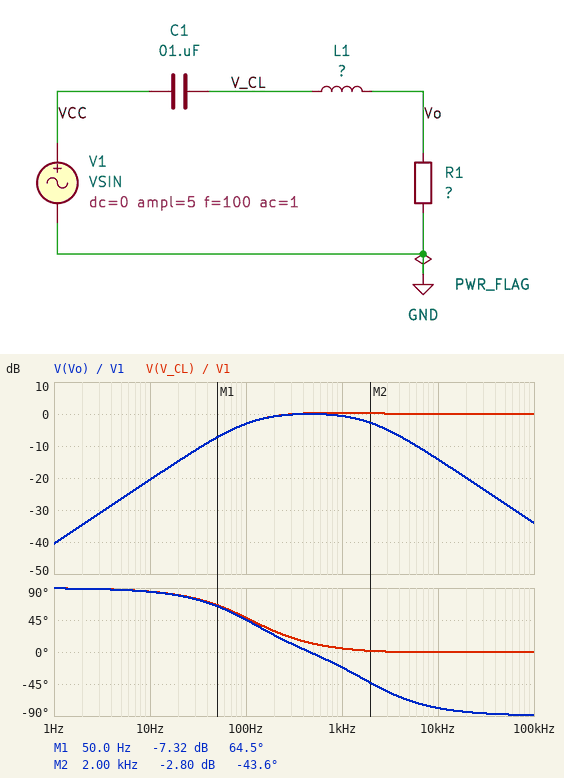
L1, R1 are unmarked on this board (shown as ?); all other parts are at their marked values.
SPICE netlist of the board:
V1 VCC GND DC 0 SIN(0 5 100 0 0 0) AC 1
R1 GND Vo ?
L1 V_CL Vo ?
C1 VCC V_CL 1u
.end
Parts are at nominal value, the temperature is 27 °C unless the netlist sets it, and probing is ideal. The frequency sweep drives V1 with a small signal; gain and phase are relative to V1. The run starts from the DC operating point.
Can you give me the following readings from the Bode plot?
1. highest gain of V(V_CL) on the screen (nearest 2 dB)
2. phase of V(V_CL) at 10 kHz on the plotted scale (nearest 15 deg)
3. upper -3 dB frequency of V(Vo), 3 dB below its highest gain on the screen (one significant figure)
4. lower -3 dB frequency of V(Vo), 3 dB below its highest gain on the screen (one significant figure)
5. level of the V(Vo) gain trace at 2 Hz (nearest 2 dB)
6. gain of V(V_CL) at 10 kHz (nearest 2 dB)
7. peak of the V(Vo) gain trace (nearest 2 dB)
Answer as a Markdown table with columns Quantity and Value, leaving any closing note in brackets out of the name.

| Quantity | Value |
|---|---|
| highest gain of V(V_CL) on the screen | 0 dB |
| phase of V(V_CL) at 10 kHz on the plotted scale | 0 deg |
| upper -3 dB frequency of V(Vo), 3 dB below its highest gain on the screen | 2 kHz |
| lower -3 dB frequency of V(Vo), 3 dB below its highest gain on the screen | 100 Hz |
| level of the V(Vo) gain trace at 2 Hz | -34 dB |
| gain of V(V_CL) at 10 kHz | 0 dB |
| peak of the V(Vo) gain trace | 0 dB |
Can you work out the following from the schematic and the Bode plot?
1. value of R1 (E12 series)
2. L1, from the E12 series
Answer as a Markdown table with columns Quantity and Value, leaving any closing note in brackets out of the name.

| Quantity | Value |
|---|---|
| value of R1 | 1.5 kΩ |
| L1, from the E12 series | 120 mH |
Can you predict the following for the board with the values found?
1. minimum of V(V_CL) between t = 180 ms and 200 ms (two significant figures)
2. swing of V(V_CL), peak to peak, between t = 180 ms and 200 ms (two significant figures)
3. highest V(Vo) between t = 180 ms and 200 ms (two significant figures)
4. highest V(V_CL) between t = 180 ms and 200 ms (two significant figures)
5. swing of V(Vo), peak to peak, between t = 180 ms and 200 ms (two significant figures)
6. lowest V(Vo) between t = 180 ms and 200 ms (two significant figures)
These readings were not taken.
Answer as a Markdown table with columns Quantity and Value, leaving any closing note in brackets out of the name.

| Quantity | Value |
|---|---|
| minimum of V(V_CL) between t = 180 ms and 200 ms | -3.5 V |
| swing of V(V_CL), peak to peak, between t = 180 ms and 200 ms | 7.0 V |
| highest V(Vo) between t = 180 ms and 200 ms | 3.5 V |
| highest V(V_CL) between t = 180 ms and 200 ms | 3.5 V |
| swing of V(Vo), peak to peak, between t = 180 ms and 200 ms | 7.0 V |
| lowest V(Vo) between t = 180 ms and 200 ms | -3.5 V |
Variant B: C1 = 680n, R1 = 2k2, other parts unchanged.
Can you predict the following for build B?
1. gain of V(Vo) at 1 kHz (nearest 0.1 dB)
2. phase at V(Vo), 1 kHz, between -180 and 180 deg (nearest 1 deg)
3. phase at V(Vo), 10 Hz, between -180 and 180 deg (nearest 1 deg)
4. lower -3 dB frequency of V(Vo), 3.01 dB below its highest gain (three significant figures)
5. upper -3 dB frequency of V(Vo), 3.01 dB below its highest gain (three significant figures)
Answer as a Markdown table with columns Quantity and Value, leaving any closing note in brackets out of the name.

| Quantity | Value |
|---|---|
| gain of V(Vo) at 1 kHz | -0.2 dB |
| phase at V(Vo), 1 kHz, between -180 and 180 deg | -13 deg |
| phase at V(Vo), 10 Hz, between -180 and 180 deg | 85 deg |
| lower -3 dB frequency of V(Vo), 3.01 dB below its highest gain | 103 Hz |
| upper -3 dB frequency of V(Vo), 3.01 dB below its highest gain | 3.02 kHz |
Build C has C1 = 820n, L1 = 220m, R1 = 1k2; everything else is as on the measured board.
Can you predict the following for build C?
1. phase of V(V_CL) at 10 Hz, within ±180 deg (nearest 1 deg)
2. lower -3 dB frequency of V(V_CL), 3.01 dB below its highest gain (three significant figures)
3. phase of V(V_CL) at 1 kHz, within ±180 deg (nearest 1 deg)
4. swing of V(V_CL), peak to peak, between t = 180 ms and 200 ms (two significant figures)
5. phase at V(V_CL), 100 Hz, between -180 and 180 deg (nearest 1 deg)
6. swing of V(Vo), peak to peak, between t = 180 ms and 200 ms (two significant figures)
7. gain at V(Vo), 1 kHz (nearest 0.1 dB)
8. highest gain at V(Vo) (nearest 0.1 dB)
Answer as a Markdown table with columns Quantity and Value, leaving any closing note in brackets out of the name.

| Quantity | Value |
|---|---|
| phase of V(V_CL) at 10 Hz, within ±180 deg | 87 deg |
| lower -3 dB frequency of V(V_CL), 3.01 dB below its highest gain | 163 Hz |
| phase of V(V_CL) at 1 kHz, within ±180 deg | 4 deg |
| swing of V(V_CL), peak to peak, between t = 180 ms and 200 ms | 5.6 V |
| phase at V(V_CL), 100 Hz, between -180 and 180 deg | 63 deg |
| swing of V(Vo), peak to peak, between t = 180 ms and 200 ms | 5.5 V |
| gain at V(Vo), 1 kHz | -3.0 dB |
| highest gain at V(Vo) | 0 dB |
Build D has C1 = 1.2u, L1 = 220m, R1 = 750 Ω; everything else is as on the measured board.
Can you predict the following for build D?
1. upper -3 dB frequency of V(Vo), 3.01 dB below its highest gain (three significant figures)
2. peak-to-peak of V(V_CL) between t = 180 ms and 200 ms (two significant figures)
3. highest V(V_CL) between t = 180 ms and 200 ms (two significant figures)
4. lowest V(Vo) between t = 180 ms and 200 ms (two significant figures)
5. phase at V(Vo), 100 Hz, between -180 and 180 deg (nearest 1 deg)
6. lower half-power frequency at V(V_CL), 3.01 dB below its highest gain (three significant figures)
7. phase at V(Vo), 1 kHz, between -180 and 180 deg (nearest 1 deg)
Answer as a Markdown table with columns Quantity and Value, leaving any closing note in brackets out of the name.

| Quantity | Value |
|---|---|
| upper -3 dB frequency of V(Vo), 3.01 dB below its highest gain | 683 Hz |
| peak-to-peak of V(V_CL) between t = 180 ms and 200 ms | 5.4 V |
| highest V(V_CL) between t = 180 ms and 200 ms | 2.7 V |
| lowest V(Vo) between t = 180 ms and 200 ms | -2.7 V |
| phase at V(Vo), 100 Hz, between -180 and 180 deg | 58 deg |
| lower half-power frequency at V(V_CL), 3.01 dB below its highest gain | 169 Hz |
| phase at V(Vo), 1 kHz, between -180 and 180 deg | -59 deg |
